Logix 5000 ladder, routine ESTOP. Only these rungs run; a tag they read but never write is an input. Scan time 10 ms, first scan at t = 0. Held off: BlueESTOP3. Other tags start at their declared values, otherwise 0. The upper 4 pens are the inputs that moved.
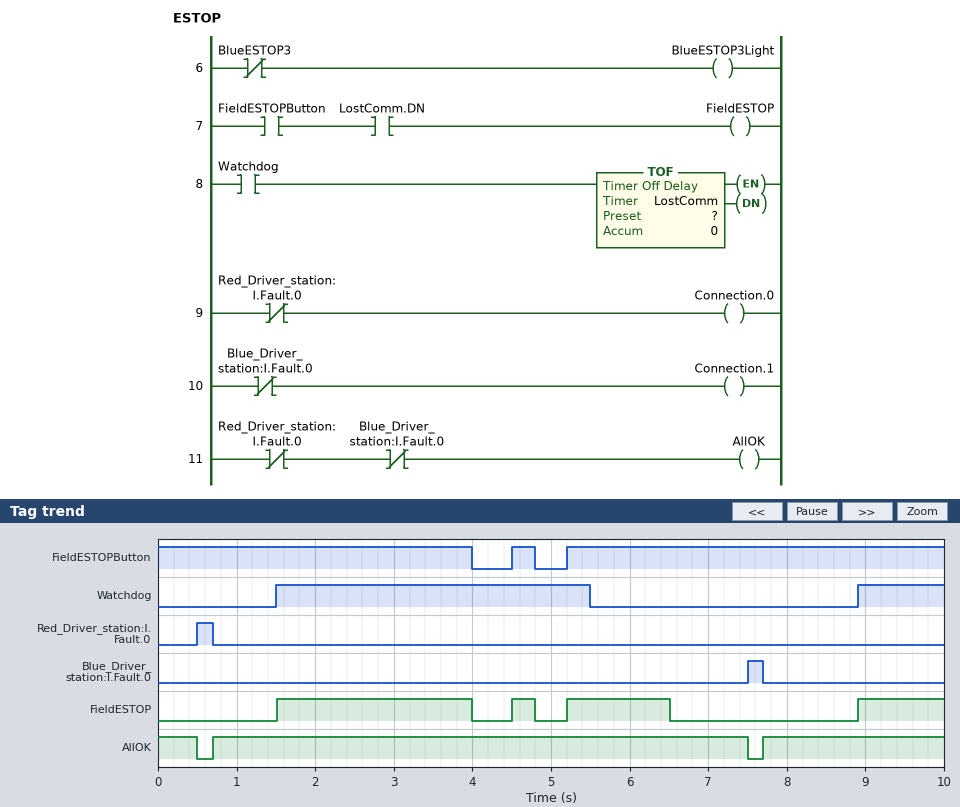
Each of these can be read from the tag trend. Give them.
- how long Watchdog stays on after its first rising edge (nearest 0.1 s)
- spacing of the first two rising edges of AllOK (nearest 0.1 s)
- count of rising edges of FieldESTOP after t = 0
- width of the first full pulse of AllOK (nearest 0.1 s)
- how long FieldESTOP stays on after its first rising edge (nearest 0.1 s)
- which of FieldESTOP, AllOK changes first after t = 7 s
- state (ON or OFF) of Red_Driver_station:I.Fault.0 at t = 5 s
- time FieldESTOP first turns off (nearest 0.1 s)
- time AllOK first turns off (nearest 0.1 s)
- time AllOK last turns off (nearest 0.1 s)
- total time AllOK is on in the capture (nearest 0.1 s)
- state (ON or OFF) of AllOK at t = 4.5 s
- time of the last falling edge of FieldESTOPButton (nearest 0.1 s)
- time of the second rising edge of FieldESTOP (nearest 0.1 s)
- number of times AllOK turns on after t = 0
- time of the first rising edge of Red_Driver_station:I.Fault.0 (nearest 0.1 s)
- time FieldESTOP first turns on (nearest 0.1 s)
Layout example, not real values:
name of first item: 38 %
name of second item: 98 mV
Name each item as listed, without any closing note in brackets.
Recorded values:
how long Watchdog stays on after its first rising edge: 4.0 s
spacing of the first two rising edges of AllOK: 7.0 s
count of rising edges of FieldESTOP after t = 0: 4
width of the first full pulse of AllOK: 6.8 s
how long FieldESTOP stays on after its first rising edge: 2.5 s
which of FieldESTOP, AllOK changes first after t = 7 s: AllOK
state (ON or OFF) of Red_Driver_station:I.Fault.0 at t = 5 s: OFF
time FieldESTOP first turns off: 4.0 s
time AllOK first turns off: 0.5 s
time AllOK last turns off: 7.5 s
total time AllOK is on in the capture: 9.6 s
state (ON or OFF) of AllOK at t = 4.5 s: ON
time of the last falling edge of FieldESTOPButton: 4.8 s
time of the second rising edge of FieldESTOP: 4.5 s
number of times AllOK turns on after t = 0: 2
time of the first rising edge of Red_Driver_station:I.Fault.0: 0.5 s
time FieldESTOP first turns on: 1.5 s
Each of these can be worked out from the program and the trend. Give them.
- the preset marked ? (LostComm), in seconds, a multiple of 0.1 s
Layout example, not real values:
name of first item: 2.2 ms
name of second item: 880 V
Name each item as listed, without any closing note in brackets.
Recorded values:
the preset marked ? (LostComm), in seconds, a multiple of 0.1 s: 1.0 s
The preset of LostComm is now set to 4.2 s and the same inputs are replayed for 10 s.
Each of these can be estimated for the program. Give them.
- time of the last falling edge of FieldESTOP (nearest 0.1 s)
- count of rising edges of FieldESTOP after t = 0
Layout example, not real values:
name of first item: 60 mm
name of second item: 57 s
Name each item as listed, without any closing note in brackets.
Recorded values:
time of the last falling edge of FieldESTOP: 4.8 s
count of rising edges of FieldESTOP after t = 0: 3
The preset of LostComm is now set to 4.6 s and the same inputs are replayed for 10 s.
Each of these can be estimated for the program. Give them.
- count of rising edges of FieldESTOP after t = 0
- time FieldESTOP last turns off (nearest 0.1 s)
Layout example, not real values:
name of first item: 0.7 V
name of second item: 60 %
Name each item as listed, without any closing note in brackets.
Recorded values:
count of rising edges of FieldESTOP after t = 0: 3
time FieldESTOP last turns off: 4.8 s
